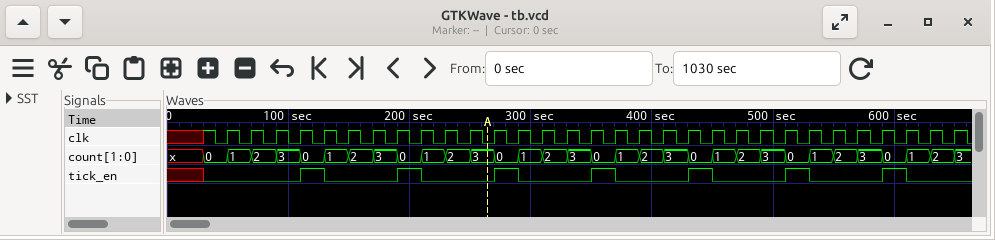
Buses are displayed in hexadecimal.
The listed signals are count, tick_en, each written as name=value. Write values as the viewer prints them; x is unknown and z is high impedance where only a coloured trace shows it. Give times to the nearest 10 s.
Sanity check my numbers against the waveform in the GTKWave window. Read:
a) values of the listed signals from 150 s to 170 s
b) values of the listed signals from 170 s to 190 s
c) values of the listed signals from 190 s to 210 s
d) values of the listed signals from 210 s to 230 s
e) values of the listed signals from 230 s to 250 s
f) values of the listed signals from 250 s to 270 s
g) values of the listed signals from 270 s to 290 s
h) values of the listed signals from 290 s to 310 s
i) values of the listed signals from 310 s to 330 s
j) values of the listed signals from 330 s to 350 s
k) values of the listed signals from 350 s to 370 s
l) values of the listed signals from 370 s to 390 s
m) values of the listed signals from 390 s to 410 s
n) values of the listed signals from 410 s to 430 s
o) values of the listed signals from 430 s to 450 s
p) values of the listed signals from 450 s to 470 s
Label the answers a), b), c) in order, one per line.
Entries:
a) count=2, tick_en=0
b) count=3, tick_en=0
c) count=0, tick_en=1
d) count=1, tick_en=0
e) count=2, tick_en=0
f) count=3, tick_en=0
g) count=0, tick_en=1
h) count=1, tick_en=0
i) count=2, tick_en=0
j) count=3, tick_en=0
k) count=0, tick_en=1
l) count=1, tick_en=0
m) count=2, tick_en=0
n) count=3, tick_en=0
o) count=0, tick_en=1
p) count=1, tick_en=0
